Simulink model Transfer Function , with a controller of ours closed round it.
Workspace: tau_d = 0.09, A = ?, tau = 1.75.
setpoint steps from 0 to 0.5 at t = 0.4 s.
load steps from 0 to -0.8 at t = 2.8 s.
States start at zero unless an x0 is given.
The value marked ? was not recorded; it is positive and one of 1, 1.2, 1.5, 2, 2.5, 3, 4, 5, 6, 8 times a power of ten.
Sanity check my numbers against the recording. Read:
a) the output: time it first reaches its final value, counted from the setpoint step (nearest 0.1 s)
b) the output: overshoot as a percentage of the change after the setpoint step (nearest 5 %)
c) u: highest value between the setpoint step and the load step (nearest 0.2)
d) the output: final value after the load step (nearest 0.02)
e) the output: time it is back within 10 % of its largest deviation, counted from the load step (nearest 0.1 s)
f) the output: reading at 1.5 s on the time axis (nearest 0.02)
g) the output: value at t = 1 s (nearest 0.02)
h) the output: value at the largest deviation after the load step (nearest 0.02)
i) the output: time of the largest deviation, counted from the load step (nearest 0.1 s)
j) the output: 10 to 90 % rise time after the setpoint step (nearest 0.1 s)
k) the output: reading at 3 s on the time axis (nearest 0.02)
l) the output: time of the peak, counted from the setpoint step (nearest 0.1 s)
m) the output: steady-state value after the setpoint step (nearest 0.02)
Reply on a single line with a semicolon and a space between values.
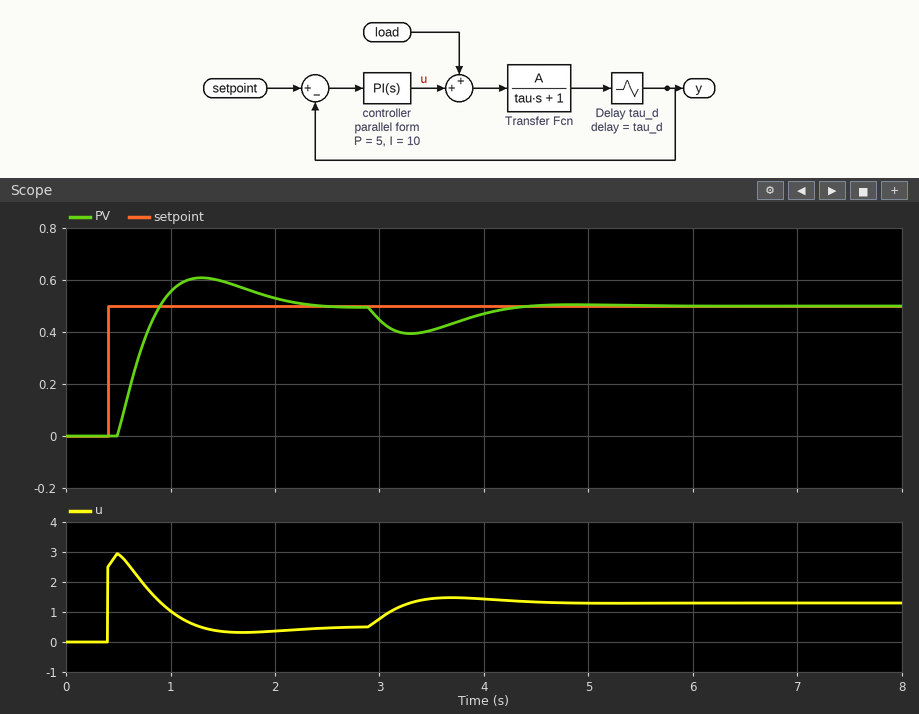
0.5 s; 20 %; 3.0; 0.50; 1.4 s; 0.60; 0.56; 0.40; 0.5 s; 0.3 s; 0.44; 0.9 s; 0.50
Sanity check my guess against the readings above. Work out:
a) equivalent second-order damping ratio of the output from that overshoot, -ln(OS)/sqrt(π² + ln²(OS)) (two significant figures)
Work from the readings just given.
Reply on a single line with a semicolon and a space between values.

0.46
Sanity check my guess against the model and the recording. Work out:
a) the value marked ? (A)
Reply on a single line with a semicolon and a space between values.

1
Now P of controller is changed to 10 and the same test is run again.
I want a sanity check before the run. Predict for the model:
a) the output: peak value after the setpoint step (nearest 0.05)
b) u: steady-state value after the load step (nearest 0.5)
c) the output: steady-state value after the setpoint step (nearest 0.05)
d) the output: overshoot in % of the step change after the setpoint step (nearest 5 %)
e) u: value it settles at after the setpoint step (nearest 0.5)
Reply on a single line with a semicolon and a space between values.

0.55; 1.5; 0.50; 10 %; 0.5
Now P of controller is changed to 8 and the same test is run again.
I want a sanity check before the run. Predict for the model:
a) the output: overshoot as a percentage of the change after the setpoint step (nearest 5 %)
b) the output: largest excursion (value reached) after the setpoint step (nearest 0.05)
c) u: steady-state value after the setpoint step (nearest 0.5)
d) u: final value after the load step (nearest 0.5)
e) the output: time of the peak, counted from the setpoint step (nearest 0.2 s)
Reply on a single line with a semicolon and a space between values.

10 %; 0.55; 0.5; 1.5; 0.6 s
